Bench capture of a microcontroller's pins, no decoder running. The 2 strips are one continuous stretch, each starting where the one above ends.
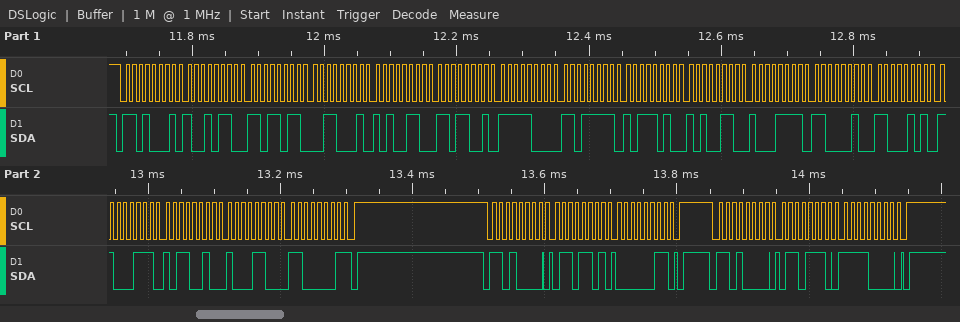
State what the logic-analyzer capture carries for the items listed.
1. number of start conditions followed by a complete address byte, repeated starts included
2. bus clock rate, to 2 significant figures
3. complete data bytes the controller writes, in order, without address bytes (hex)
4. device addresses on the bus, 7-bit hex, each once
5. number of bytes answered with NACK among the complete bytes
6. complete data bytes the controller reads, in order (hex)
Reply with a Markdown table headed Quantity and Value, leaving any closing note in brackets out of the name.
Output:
| Quantity | Value |
|---|---|
| number of start conditions followed by a complete address byte, repeated starts included | 3 |
| bus clock rate, to 2 significant figures | 100 kHz |
| complete data bytes the controller writes, in order, without address bytes | 6D 03 6E F0 |
| device addresses on the bus, 7-bit hex, each once | 0x68 |
| number of bytes answered with NACK among the complete bytes | 1 |
| complete data bytes the controller reads, in order | 96 DB 31 A6 D9 F8 DF BA A6 8F C2 C5 C7 B2 8C C1 |
